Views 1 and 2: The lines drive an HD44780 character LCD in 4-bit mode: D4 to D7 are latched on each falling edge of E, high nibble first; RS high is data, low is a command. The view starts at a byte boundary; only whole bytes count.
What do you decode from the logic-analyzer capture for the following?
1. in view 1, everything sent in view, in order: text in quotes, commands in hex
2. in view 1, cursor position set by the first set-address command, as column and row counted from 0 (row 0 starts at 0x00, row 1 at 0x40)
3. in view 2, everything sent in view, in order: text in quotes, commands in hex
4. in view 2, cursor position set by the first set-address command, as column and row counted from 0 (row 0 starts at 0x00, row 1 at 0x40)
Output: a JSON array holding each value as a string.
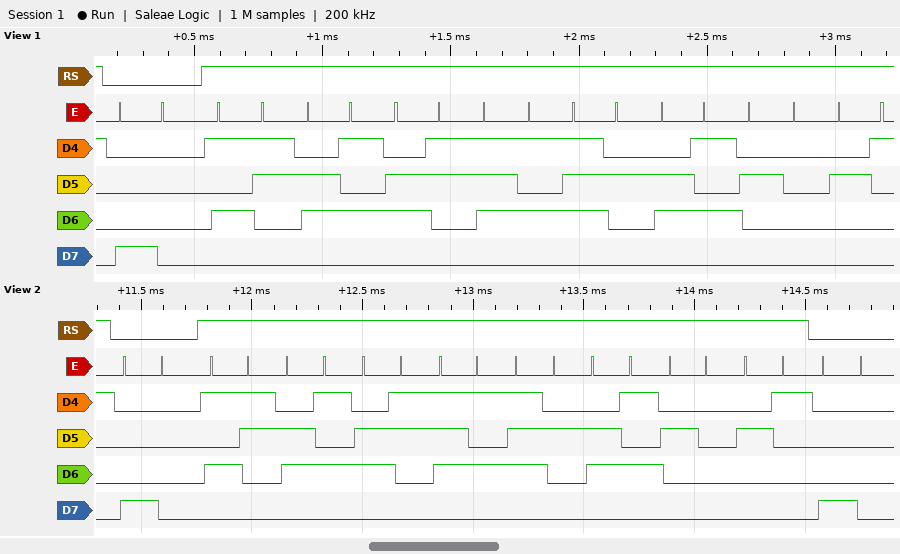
["0x80 \"Secure !\"", "column 0, row 0", "0x80 \"Secure !\" 0x80", "column 0, row 0"]
